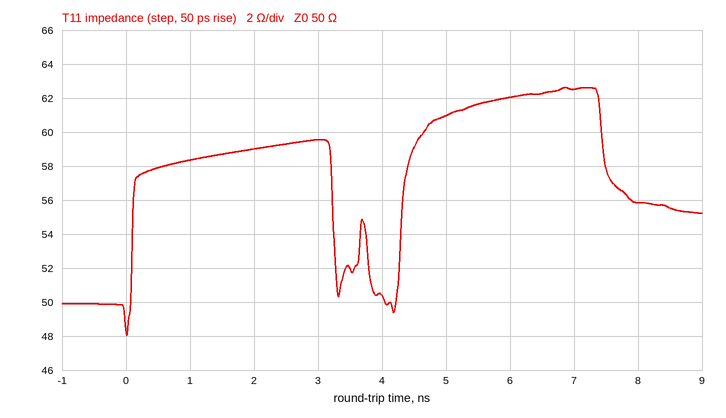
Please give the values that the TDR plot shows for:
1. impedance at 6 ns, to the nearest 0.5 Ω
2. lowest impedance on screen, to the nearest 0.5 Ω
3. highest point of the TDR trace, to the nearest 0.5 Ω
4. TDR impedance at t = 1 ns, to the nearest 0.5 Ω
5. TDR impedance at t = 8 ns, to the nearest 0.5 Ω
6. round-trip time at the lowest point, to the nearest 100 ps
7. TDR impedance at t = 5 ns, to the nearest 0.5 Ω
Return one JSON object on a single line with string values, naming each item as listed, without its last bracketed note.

{"impedance at 6 ns, to the nearest 0.5 Ω": "62.0 Ω", "lowest impedance on screen, to the nearest 0.5 Ω": "48.0 Ω", "highest point of the TDR trace, to the nearest 0.5 Ω": "62.5 Ω", "TDR impedance at t = 1 ns, to the nearest 0.5 Ω": "58.5 Ω", "TDR impedance at t = 8 ns, to the nearest 0.5 Ω": "56.0 Ω", "round-trip time at the lowest point, to the nearest 100 ps": "0.0 ns", "TDR impedance at t = 5 ns, to the nearest 0.5 Ω": "61.0 Ω"}
